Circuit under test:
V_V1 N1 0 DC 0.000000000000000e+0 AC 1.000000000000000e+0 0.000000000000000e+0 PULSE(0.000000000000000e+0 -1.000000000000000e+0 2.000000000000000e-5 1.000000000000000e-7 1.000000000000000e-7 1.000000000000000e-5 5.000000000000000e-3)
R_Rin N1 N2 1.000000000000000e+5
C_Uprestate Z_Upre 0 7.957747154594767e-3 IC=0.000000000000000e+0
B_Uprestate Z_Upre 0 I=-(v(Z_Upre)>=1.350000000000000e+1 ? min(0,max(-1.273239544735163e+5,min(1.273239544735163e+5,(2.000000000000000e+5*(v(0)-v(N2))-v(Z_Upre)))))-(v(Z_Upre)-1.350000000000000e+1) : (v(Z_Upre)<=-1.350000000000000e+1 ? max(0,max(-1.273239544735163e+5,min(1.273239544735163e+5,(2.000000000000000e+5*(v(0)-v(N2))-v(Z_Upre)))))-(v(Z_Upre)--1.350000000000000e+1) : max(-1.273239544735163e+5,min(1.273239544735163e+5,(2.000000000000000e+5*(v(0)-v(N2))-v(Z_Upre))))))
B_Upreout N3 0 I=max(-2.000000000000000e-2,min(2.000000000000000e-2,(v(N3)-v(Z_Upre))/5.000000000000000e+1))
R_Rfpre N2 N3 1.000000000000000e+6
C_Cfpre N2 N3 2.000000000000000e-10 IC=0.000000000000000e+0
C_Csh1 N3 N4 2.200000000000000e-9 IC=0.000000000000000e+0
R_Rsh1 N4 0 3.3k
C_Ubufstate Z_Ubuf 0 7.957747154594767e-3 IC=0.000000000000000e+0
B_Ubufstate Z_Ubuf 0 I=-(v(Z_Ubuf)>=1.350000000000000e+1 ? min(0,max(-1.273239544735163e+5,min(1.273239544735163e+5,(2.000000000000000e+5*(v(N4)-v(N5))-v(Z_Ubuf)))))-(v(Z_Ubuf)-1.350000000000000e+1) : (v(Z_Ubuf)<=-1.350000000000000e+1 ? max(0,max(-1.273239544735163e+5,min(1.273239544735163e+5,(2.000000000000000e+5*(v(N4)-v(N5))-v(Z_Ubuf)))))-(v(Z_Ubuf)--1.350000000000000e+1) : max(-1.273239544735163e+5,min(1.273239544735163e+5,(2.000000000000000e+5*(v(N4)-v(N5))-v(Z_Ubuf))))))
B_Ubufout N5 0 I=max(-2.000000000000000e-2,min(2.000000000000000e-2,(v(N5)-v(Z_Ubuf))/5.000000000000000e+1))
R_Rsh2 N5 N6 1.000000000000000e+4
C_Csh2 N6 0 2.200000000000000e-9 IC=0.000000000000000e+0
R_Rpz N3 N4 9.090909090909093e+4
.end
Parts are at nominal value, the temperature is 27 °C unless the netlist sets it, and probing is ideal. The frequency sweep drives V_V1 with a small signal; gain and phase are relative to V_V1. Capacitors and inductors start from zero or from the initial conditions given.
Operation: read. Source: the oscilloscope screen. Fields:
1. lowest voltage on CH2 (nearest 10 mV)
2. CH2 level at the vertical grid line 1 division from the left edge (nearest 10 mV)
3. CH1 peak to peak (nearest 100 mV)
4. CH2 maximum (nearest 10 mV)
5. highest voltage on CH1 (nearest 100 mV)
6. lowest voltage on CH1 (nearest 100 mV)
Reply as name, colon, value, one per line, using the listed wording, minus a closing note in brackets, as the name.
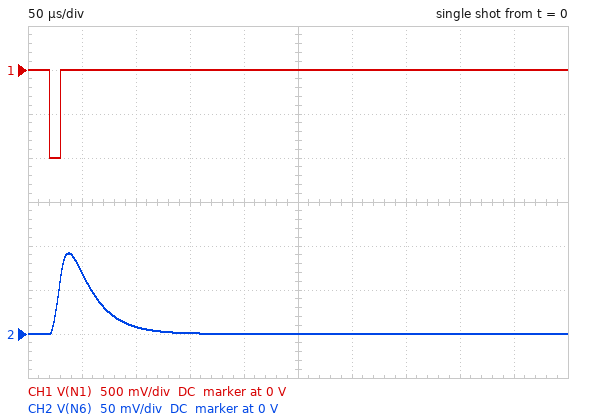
lowest voltage on CH2: 0 V
CH2 level at the vertical grid line 1 division from the left edge: 70 mV
CH1 peak to peak: 1.0 V
CH2 maximum: 90 mV
highest voltage on CH1: 0 V
lowest voltage on CH1: -1.0 V
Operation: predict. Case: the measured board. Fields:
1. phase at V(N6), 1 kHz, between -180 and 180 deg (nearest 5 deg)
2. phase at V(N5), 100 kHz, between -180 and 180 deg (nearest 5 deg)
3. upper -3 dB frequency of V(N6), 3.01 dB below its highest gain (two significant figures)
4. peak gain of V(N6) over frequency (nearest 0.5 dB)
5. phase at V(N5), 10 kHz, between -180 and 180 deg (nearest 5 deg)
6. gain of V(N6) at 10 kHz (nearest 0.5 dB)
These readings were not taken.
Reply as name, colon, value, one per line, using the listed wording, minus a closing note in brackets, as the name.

phase at V(N6), 1 kHz, between -180 and 180 deg: 170 deg
phase at V(N5), 100 kHz, between -180 and 180 deg: 100 deg
upper -3 dB frequency of V(N6), 3.01 dB below its highest gain: 6.6 kHz
peak gain of V(N6) over frequency: -9.0 dB
phase at V(N5), 10 kHz, between -180 and 180 deg: 155 deg
gain of V(N6) at 10 kHz: -14.5 dB
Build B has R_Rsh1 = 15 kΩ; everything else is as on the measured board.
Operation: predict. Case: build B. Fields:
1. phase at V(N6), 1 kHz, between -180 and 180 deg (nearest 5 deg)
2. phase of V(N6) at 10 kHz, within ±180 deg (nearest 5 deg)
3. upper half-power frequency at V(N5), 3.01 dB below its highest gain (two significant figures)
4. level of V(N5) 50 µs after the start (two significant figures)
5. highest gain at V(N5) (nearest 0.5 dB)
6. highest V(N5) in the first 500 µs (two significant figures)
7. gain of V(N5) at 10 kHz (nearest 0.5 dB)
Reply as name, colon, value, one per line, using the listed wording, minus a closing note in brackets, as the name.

phase at V(N6), 1 kHz, between -180 and 180 deg: 160 deg
phase of V(N6) at 10 kHz, within ±180 deg: 65 deg
upper half-power frequency at V(N5), 3.01 dB below its highest gain: 5.6 kHz
level of V(N5) 50 µs after the start: 210 mV
highest gain at V(N5): 3.0 dB
highest V(N5) in the first 500 µs: 420 mV
gain of V(N5) at 10 kHz: -3.0 dB
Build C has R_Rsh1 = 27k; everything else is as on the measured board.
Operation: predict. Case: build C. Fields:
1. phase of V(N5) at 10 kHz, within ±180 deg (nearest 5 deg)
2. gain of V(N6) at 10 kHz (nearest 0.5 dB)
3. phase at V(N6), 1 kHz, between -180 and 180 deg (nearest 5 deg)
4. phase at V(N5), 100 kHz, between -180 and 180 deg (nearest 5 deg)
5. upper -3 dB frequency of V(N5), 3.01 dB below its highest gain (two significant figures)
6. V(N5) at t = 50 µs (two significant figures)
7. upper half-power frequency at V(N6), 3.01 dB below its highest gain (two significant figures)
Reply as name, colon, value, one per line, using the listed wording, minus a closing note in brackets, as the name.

phase of V(N5) at 10 kHz, within ±180 deg: 110 deg
gain of V(N6) at 10 kHz: -7.0 dB
phase at V(N6), 1 kHz, between -180 and 180 deg: 155 deg
phase at V(N5), 100 kHz, between -180 and 180 deg: 90 deg
upper -3 dB frequency of V(N5), 3.01 dB below its highest gain: 3.5 kHz
V(N5) at t = 50 µs: 290 mV
upper half-power frequency at V(N6), 3.01 dB below its highest gain: 2.9 kHz
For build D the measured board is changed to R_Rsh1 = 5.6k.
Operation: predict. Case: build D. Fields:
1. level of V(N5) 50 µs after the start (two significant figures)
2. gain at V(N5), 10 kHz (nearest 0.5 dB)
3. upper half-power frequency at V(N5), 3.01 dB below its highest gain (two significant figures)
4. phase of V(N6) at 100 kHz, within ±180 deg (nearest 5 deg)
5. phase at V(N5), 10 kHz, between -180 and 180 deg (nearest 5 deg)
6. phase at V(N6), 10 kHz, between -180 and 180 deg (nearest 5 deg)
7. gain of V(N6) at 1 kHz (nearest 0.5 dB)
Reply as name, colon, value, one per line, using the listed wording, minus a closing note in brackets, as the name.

level of V(N5) 50 µs after the start: 61 mV
gain at V(N5), 10 kHz: -6.5 dB
upper half-power frequency at V(N5), 3.01 dB below its highest gain: 14 kHz
phase of V(N6) at 100 kHz, within ±180 deg: 10 deg
phase at V(N5), 10 kHz, between -180 and 180 deg: 145 deg
phase at V(N6), 10 kHz, between -180 and 180 deg: 90 deg
gain of V(N6) at 1 kHz: -5.0 dB
